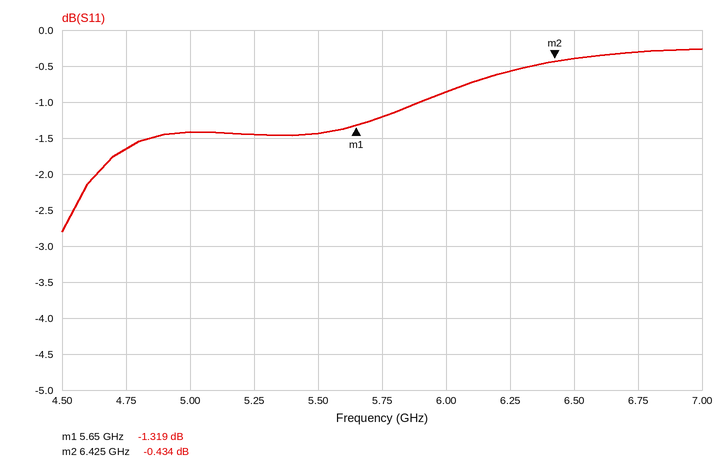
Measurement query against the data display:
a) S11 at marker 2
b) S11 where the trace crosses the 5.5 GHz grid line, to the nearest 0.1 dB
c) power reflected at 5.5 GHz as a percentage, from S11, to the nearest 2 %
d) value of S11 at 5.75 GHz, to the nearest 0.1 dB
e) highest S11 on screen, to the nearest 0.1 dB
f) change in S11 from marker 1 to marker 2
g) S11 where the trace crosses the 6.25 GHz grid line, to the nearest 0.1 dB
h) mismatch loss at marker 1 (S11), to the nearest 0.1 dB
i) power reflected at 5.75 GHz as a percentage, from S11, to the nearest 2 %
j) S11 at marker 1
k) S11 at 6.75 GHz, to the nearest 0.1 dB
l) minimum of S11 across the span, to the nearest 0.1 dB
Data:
-0.434 dB
-1.4 dB
72 %
-1.2 dB
-0.3 dB
0.885 dB
-0.6 dB
5.8 dB
76 %
-1.319 dB
-0.3 dB
-2.8 dB
